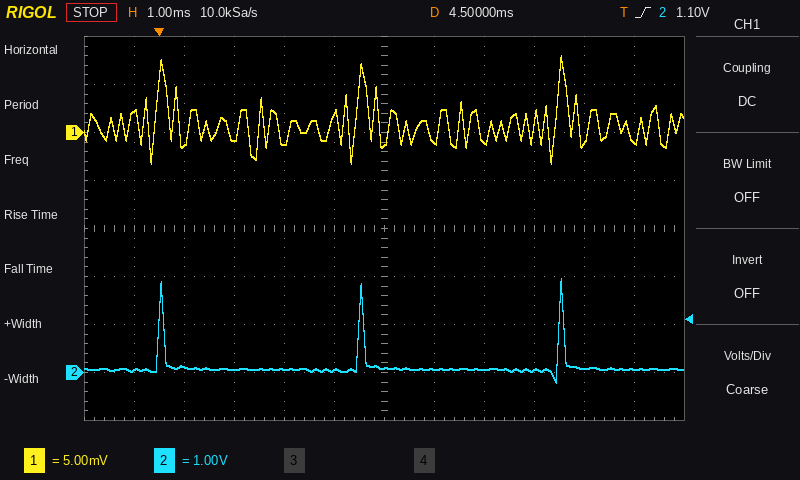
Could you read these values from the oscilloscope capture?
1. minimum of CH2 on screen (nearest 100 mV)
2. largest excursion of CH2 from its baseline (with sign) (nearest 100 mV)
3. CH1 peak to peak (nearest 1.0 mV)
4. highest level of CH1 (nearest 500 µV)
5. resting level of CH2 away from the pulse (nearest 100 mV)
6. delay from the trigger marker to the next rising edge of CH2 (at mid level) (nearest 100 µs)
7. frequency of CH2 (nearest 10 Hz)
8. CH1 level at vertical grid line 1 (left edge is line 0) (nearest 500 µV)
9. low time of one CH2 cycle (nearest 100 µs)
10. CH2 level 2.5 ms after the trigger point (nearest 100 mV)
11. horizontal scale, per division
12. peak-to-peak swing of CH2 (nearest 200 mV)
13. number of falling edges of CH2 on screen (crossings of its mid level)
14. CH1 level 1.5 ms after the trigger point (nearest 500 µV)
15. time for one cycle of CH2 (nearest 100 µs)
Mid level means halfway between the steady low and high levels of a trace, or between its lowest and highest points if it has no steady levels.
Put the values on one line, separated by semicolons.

-200 mV; +1.9 V; 11.0 mV; 8.0 mV; 100 mV; 4.0 ms; 250 Hz; 2.0 mV; 3.9 ms; 100 mV; 1 ms; 2.2 V; 3; -500 µV; 4.0 ms
